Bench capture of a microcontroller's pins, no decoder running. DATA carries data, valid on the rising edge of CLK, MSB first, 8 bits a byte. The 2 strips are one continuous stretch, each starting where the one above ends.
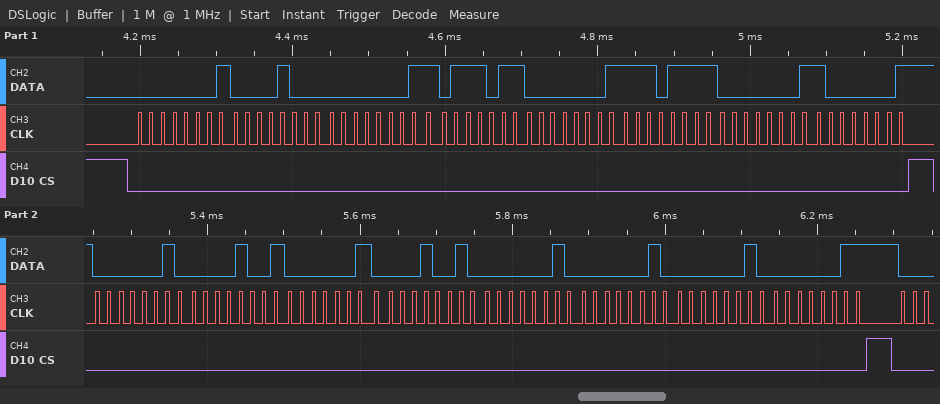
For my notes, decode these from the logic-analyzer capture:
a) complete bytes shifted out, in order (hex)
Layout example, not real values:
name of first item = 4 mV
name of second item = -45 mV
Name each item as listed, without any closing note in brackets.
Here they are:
complete bytes shifted out, in order = 01 08 01 BB 01 EF 01 81 02 09 02 12 02 02 02 03
